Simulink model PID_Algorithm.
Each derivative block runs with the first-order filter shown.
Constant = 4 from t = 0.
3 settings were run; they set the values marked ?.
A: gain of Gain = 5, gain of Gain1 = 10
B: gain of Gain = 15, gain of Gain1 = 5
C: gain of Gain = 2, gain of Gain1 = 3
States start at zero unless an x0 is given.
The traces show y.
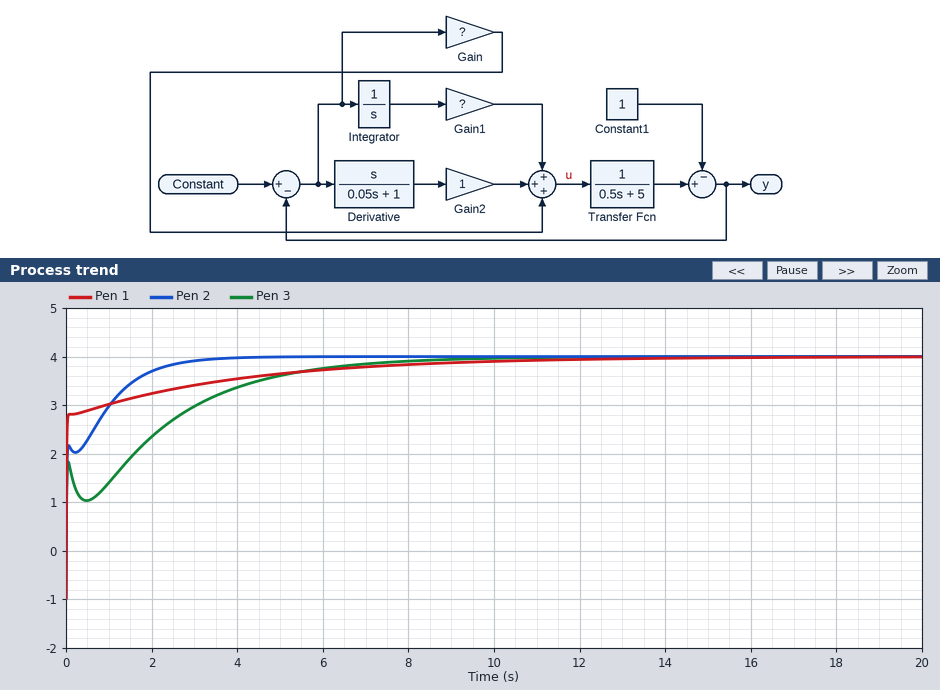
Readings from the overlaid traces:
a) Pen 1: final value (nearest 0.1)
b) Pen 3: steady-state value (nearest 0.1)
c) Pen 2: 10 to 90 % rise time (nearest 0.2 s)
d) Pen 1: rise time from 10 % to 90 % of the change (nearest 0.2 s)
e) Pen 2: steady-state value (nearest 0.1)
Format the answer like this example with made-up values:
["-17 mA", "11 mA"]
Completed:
["4.0", "4.0", "1.6 s", "3.6 s", "4.0"]
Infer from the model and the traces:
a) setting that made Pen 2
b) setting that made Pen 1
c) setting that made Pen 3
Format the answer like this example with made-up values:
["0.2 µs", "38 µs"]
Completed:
["A", "B", "C"]
